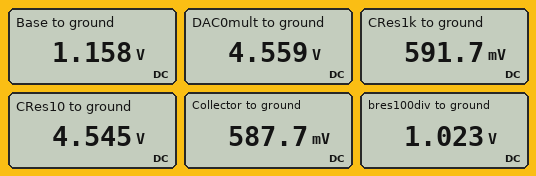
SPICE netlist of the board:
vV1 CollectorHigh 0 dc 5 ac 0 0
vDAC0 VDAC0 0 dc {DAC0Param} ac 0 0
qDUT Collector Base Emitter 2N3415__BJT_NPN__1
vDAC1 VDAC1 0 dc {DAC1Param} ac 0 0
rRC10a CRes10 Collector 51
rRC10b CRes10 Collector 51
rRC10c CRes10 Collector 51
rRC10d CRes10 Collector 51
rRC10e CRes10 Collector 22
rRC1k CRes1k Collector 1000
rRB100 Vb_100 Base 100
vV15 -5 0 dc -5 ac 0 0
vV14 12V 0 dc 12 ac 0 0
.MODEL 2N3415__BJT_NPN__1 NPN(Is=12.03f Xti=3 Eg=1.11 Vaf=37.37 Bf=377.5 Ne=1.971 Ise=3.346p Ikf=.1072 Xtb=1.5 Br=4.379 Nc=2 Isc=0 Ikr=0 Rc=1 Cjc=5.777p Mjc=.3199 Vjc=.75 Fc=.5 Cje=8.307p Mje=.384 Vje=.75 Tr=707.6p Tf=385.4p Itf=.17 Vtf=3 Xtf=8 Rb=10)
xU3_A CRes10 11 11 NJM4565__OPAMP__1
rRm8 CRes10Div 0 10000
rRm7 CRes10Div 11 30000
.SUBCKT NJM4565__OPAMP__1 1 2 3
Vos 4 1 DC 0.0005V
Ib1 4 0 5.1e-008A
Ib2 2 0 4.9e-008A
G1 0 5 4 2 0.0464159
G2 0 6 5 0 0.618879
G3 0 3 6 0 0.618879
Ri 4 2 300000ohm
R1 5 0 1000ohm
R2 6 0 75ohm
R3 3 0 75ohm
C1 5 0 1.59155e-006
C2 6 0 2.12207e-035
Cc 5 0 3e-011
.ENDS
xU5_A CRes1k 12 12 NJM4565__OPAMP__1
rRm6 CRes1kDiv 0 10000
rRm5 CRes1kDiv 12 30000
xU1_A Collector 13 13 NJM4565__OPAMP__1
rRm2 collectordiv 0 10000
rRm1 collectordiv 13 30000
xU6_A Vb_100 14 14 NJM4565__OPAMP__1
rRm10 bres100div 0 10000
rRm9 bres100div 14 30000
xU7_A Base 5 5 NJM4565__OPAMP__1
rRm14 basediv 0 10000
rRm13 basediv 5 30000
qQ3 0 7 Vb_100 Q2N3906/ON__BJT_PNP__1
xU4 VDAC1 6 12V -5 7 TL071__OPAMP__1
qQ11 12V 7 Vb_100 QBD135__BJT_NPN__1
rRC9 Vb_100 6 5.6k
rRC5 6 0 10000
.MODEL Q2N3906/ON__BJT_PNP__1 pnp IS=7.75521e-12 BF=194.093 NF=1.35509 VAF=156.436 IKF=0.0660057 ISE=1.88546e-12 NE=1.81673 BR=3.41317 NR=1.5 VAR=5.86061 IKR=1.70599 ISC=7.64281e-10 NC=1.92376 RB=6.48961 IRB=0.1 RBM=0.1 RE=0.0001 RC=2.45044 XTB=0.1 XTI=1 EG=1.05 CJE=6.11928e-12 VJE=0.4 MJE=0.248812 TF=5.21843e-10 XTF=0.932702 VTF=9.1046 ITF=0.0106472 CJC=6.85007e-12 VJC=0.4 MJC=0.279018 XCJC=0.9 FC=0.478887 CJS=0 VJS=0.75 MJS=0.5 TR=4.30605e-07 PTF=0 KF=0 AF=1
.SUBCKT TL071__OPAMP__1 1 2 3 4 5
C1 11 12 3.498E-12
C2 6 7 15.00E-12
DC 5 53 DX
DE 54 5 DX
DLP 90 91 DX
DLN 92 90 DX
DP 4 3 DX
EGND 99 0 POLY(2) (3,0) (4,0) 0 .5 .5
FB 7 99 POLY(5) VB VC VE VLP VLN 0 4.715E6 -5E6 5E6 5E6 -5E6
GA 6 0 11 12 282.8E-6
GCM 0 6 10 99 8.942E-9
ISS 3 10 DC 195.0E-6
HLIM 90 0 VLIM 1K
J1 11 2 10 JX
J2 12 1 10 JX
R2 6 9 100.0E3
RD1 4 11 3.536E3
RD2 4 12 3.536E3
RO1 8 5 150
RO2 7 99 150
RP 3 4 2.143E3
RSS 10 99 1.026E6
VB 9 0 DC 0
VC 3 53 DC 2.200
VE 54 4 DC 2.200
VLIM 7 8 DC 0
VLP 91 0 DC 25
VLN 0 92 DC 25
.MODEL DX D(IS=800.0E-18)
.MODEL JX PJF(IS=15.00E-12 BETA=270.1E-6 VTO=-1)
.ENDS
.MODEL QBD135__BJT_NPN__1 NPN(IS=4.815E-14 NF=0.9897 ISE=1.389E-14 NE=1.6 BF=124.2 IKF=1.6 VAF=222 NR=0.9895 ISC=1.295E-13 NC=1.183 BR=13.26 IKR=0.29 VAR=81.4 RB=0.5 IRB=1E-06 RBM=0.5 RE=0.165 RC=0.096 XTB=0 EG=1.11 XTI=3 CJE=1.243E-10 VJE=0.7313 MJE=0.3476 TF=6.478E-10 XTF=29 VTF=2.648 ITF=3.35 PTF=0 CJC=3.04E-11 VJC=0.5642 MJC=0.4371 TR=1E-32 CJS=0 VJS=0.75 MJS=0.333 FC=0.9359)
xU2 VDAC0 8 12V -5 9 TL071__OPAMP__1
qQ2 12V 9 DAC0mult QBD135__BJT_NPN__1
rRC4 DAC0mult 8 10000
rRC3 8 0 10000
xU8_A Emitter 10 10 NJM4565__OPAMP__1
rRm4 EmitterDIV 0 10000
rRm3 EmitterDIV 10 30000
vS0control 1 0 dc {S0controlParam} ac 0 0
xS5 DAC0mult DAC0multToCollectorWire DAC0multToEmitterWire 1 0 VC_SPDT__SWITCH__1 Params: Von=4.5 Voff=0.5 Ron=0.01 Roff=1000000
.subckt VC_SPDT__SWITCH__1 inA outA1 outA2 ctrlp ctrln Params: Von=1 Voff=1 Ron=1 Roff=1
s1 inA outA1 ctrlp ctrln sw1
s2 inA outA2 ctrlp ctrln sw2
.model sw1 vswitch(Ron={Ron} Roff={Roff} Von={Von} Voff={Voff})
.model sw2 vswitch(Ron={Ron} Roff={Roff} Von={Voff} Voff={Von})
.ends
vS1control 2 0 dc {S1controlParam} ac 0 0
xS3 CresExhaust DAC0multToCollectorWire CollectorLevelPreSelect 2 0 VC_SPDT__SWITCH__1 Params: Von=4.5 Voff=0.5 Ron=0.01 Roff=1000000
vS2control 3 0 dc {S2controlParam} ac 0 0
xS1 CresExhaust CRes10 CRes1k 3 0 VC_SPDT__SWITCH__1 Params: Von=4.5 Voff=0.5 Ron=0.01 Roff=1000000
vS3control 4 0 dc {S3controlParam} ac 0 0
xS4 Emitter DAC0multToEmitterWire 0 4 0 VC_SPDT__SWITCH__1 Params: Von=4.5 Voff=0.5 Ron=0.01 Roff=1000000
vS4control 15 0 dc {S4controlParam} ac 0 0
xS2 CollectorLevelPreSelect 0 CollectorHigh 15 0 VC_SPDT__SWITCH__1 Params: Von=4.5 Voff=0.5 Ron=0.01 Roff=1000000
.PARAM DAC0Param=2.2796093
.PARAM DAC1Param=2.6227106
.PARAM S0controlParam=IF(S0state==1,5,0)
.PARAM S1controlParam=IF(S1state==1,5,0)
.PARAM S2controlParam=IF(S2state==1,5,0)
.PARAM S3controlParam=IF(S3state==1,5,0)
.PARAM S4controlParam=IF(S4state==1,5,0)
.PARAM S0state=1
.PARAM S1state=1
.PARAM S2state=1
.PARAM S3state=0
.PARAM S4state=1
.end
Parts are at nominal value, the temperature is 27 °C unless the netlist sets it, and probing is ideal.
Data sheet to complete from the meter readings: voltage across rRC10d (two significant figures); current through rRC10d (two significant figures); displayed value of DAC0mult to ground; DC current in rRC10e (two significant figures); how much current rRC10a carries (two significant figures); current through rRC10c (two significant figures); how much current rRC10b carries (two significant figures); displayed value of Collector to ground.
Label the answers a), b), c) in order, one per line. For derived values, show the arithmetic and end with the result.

a) 4.545 V - 587.7 mV = 4.0 V
b) (4.545 V - 587.7 mV) / 51 Ω = 78 mA
c) 4.559 V
d) (4.545 V - 587.7 mV) / 22 Ω = 180 mA
e) (4.545 V - 587.7 mV) / 51 Ω = 78 mA
f) (4.545 V - 587.7 mV) / 51 Ω = 78 mA
g) (4.545 V - 587.7 mV) / 51 Ω = 78 mA
h) 587.7 mV
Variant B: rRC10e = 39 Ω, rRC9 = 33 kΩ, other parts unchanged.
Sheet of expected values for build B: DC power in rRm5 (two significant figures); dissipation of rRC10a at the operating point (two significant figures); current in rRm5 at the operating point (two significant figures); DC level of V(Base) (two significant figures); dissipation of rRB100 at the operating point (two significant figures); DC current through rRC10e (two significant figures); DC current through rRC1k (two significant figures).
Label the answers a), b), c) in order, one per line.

a) 4.6 µW
b) 320 mW
c) 12 µA
d) 1.7 V
e) 650 mW
f) 100 mA
g) 4.1 µA
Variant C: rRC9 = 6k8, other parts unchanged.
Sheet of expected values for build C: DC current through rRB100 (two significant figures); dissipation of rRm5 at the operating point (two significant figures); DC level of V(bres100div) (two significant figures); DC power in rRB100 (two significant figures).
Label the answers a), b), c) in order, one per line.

a) 32 mA
b) 6.5 µW
c) 1.1 V
d) 100 mW
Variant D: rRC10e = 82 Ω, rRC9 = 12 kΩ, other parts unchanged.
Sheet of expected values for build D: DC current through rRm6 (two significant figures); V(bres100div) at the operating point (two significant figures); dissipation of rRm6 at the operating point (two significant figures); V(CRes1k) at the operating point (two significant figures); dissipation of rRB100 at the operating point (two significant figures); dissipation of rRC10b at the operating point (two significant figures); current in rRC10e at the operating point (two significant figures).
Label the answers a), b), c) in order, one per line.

a) 11 µA
b) 1.4 V
c) 1.3 µW
d) 450 mV
e) 200 mW
f) 330 mW
g) 50 mA
